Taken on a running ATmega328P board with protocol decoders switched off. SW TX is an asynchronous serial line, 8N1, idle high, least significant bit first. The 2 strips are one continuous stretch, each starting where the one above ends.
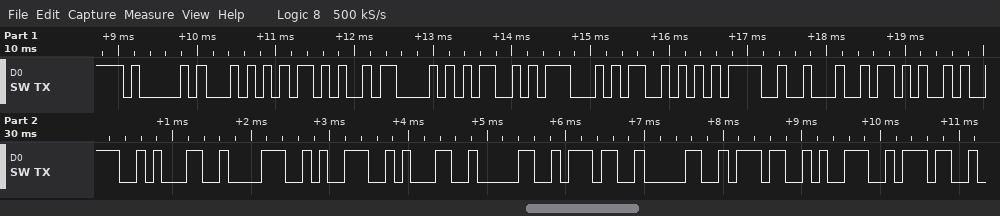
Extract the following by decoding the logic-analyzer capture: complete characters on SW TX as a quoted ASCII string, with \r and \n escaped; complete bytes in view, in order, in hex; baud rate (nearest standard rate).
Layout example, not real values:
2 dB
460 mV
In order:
"AT+CMGS=\"+91891070797"
41 54 2B 43 4D 47 53 3D 22 2B 39 31 38 39 31 30 37 30 37 39 37
9600 baud
